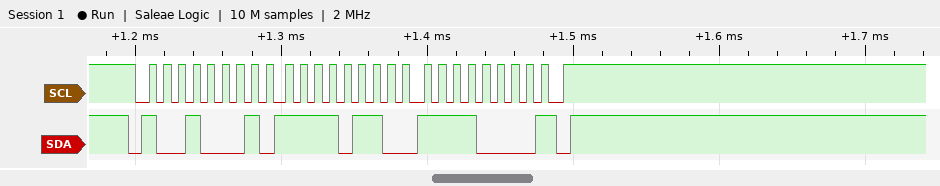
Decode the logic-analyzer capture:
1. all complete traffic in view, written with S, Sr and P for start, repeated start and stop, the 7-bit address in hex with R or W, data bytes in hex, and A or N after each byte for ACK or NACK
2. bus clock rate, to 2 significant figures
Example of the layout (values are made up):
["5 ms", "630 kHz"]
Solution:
["S 48R A F6 A F0 N P", "100 kHz"]
